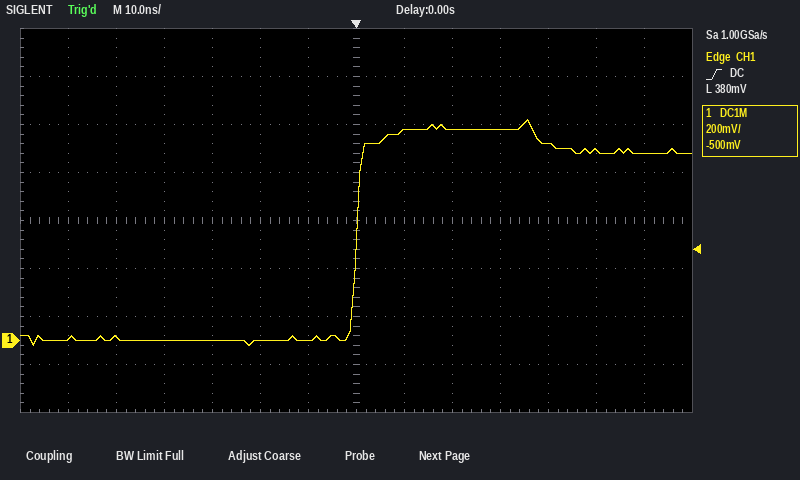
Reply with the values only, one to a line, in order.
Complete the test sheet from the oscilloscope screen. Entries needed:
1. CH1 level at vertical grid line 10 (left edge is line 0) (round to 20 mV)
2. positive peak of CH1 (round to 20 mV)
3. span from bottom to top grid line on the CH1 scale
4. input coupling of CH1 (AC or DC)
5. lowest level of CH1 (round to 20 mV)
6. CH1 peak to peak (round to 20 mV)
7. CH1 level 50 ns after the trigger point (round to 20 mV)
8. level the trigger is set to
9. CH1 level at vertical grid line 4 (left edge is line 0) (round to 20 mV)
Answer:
880 mV
920 mV
1.6 V
DC
-20 mV
940 mV
800 mV
380 mV
0 mV
